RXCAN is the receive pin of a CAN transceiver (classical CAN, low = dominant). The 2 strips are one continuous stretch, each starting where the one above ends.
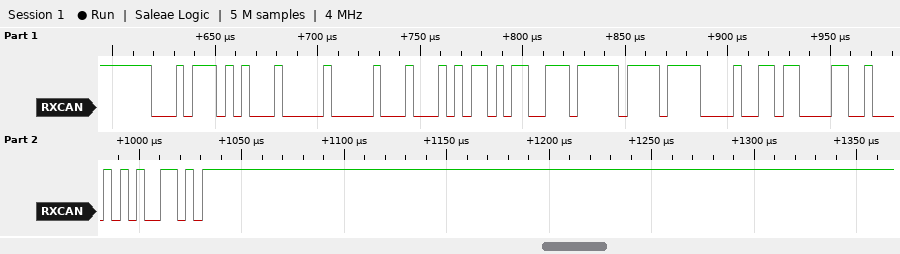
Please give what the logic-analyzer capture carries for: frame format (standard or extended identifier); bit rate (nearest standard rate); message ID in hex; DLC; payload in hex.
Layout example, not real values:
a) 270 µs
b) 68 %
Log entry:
a) standard
b) 250 kbit/s
c) 0x175
d) 8
e) 00 22 B5 9D FF 78 4D 86
